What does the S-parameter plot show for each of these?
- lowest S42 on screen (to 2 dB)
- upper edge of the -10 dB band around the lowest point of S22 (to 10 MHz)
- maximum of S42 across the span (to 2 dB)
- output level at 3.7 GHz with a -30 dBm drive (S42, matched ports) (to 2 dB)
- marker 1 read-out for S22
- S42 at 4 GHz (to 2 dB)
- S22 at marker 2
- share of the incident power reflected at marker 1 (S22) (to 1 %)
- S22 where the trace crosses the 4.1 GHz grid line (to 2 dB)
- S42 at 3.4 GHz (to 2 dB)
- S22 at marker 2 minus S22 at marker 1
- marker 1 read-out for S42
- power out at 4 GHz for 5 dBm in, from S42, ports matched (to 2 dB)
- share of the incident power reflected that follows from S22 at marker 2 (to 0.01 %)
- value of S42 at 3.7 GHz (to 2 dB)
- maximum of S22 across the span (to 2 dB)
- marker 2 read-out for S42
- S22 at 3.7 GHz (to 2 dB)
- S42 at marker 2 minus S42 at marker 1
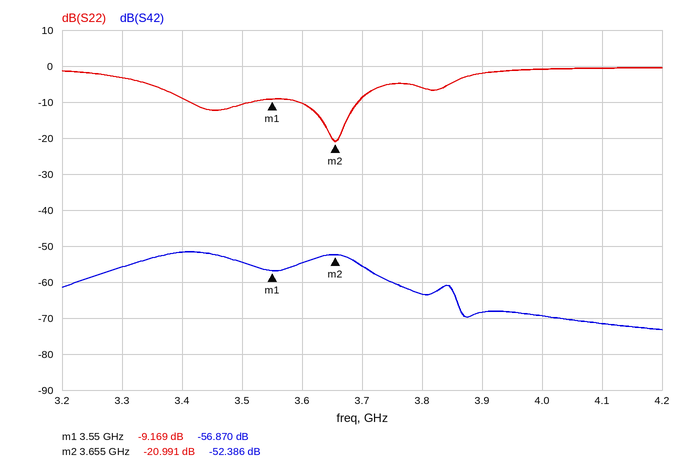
-74 dB
3.69 GHz
-52 dB
-86 dBm
-9.169 dB
-70 dB
-20.991 dB
12 %
0 dB
-52 dB
-11.822 dB
-56.870 dB
-64 dBm
0.80 %
-56 dB
0 dB
-52.386 dB
-8 dB
4.484 dB
